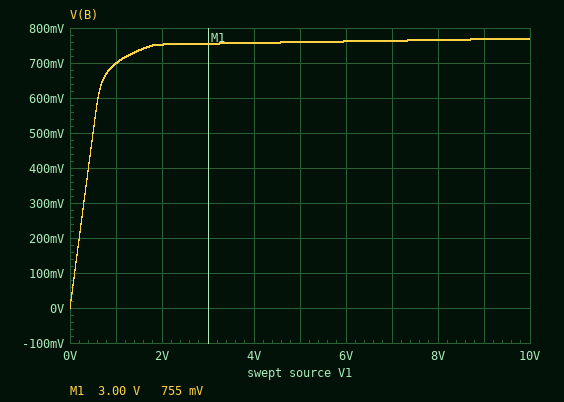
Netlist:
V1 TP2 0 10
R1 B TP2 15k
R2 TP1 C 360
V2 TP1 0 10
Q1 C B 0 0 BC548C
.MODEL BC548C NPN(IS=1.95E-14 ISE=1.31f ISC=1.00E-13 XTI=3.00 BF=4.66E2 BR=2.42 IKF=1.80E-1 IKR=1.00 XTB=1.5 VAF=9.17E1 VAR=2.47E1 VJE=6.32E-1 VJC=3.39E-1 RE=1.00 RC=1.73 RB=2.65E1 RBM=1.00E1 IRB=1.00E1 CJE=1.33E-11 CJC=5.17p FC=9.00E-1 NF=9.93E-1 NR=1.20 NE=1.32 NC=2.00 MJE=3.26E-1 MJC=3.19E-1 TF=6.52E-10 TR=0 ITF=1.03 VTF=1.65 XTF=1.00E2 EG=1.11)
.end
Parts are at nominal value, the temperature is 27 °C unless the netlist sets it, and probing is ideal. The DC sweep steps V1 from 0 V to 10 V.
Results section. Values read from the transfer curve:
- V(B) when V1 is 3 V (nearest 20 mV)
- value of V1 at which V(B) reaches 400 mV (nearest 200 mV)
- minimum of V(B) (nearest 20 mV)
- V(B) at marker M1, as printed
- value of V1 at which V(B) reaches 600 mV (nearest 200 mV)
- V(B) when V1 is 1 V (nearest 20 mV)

760 mV
400 mV
0 V
755 mV
600 mV
700 mV
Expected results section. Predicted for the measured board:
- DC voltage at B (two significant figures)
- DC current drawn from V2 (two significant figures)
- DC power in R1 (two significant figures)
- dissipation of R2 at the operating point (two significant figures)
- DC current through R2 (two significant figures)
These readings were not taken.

770 mV
28 mA
5.7 mW
280 mW
28 mA
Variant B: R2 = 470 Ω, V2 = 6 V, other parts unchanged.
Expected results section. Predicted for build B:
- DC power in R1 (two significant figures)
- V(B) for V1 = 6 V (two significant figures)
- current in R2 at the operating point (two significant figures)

5.7 mW
730 mV
13 mA
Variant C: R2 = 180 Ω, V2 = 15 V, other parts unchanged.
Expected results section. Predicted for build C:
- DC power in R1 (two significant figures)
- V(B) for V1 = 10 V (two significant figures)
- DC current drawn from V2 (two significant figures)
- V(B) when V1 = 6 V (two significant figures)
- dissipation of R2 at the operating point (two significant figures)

5.6 mW
860 mV
82 mA
850 mV
1.2 W
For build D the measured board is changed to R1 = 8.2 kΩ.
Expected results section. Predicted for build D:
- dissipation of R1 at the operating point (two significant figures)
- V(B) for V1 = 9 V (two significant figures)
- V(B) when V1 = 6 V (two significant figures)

10 mW
780 mV
770 mV
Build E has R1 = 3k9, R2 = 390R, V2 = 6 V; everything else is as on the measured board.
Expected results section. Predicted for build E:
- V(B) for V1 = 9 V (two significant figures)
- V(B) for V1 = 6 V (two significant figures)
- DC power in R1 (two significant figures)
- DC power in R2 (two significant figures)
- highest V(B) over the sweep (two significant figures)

790 mV
770 mV
22 mW
94 mW
800 mV
